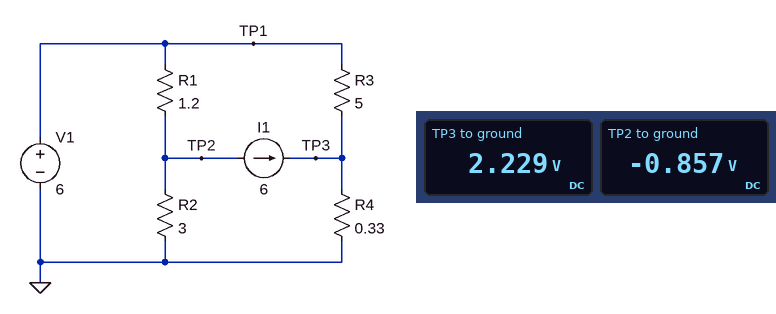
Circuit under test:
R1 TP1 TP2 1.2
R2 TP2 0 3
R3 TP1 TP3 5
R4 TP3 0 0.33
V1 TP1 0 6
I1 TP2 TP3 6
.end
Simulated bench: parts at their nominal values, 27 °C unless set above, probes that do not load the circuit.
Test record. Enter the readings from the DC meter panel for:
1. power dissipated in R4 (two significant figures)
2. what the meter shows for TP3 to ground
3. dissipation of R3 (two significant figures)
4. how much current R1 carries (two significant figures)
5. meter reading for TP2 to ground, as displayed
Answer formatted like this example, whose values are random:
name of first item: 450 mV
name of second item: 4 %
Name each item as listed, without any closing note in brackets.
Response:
power dissipated in R4: 15 W
what the meter shows for TP3 to ground: 2.229 V
dissipation of R3: 2.8 W
how much current R1 carries: 5.7 A
meter reading for TP2 to ground, as displayed: -0.857 V
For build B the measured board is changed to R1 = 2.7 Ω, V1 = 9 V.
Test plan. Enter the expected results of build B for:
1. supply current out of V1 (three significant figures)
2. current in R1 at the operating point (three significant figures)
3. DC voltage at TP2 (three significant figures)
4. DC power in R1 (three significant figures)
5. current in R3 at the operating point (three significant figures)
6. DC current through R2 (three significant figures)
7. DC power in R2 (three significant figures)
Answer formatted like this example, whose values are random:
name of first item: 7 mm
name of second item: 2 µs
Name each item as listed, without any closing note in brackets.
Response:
supply current out of V1: 6.05 A
current in R1 at the operating point: 4.74 A
DC voltage at TP2: -3.79 V
DC power in R1: 60.6 W
current in R3 at the operating point: 1.32 A
DC current through R2: 1.26 A
DC power in R2: 4.79 W
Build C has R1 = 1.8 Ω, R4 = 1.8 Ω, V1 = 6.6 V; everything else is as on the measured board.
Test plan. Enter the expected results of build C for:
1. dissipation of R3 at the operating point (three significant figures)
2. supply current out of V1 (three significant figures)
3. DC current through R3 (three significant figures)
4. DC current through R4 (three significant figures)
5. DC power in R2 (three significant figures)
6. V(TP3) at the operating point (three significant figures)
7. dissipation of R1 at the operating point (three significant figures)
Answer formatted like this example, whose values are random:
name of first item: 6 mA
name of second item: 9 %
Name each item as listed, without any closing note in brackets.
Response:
dissipation of R3 at the operating point: 1.91 W
supply current out of V1: 4.51 A
DC current through R3: 618 mA
DC current through R4: 5.38 A
DC power in R2: 2.30 W
V(TP3) at the operating point: 9.69 V
dissipation of R1 at the operating point: 47.3 W
